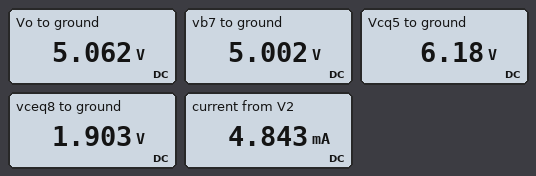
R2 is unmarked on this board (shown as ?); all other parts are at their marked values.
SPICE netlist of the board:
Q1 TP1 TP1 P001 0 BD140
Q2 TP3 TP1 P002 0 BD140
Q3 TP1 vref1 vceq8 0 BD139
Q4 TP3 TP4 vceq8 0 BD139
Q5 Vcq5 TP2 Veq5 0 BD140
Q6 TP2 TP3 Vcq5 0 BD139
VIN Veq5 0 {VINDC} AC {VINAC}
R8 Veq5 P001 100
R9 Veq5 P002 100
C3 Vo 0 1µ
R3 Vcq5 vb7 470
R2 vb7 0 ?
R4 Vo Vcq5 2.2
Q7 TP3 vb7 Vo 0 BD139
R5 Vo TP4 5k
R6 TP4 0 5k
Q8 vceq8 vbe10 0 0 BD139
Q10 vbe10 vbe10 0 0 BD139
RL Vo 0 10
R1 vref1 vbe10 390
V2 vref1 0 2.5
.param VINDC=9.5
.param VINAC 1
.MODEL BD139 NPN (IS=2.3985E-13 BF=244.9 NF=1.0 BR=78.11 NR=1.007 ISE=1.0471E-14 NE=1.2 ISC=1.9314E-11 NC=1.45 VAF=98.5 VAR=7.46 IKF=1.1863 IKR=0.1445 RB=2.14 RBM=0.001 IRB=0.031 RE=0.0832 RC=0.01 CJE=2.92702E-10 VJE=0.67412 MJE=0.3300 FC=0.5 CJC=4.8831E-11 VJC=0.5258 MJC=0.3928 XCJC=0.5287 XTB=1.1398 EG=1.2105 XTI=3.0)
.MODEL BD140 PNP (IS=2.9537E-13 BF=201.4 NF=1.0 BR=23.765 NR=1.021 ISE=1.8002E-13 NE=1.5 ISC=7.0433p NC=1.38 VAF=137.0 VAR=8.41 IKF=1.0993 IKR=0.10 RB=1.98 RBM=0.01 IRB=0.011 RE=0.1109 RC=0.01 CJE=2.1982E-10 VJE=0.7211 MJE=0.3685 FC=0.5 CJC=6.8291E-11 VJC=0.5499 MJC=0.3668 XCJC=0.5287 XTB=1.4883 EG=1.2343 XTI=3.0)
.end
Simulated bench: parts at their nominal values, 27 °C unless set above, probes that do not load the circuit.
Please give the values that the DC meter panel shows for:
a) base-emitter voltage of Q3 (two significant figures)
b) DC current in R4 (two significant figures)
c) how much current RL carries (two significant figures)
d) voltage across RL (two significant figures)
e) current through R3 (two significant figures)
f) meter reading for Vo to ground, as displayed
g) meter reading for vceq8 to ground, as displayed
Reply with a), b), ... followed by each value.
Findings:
a) 600 mV
b) 510 mA
c) 510 mA
d) 5.1 V
e) 2.5 mA
f) 5.062 V
g) 1.903 V
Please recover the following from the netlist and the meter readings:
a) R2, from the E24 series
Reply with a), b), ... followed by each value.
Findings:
a) 2 kΩ
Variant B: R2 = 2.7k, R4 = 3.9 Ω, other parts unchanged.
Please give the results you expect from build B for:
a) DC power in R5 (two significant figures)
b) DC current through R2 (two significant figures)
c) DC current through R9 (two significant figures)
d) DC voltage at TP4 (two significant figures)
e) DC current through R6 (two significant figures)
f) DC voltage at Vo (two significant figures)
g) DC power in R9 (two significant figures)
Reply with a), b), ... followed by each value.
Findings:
a) 610 µW
b) 1.5 mA
c) 4.8 mA
d) 1.7 V
e) 350 µA
f) 3.5 V
g) 2.3 mW
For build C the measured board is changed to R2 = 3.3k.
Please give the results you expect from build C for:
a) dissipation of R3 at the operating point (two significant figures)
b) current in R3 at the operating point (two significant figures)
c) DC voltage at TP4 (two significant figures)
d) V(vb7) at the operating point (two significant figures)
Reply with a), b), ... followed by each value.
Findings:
a) 1.3 mW
b) 1.6 mA
c) 2.5 V
d) 5.4 V
